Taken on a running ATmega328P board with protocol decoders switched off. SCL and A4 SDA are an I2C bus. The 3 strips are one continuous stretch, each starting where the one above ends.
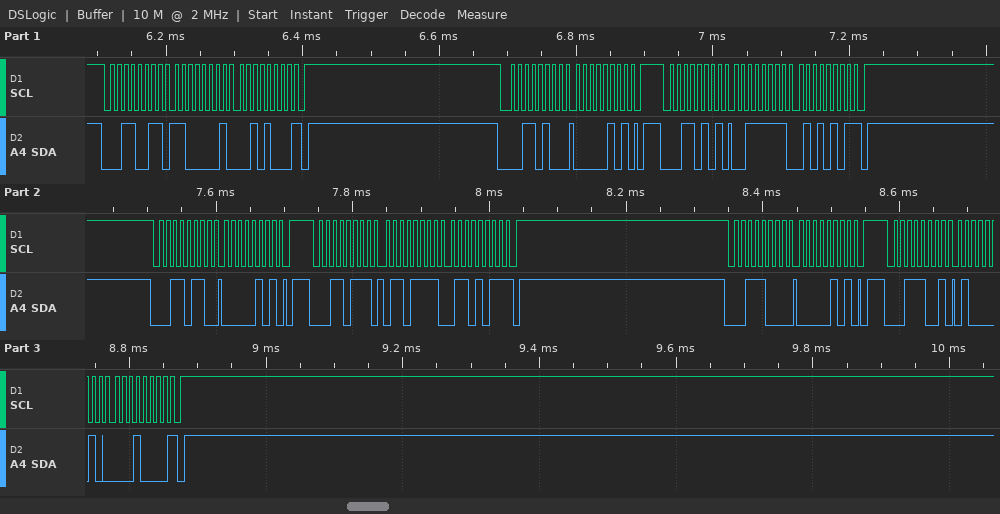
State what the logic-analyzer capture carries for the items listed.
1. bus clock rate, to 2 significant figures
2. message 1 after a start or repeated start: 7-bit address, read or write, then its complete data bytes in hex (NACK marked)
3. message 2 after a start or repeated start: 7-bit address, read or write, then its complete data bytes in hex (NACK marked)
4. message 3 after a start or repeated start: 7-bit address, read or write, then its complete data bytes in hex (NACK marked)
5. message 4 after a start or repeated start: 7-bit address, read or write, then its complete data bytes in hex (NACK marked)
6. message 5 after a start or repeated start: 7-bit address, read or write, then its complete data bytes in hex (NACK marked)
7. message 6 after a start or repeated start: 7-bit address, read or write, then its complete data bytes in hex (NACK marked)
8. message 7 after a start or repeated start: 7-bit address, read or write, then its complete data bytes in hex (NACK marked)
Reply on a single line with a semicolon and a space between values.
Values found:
100 kHz; 0x19 read: C1 28 NACK; 0x1A write: 05; 0x1A read: 3F 55 NACK; 0x1B write: 05; 0x1B read: 6F 6B NACK; 0x1C write: 05; 0x1C read: 42 10 NACK
